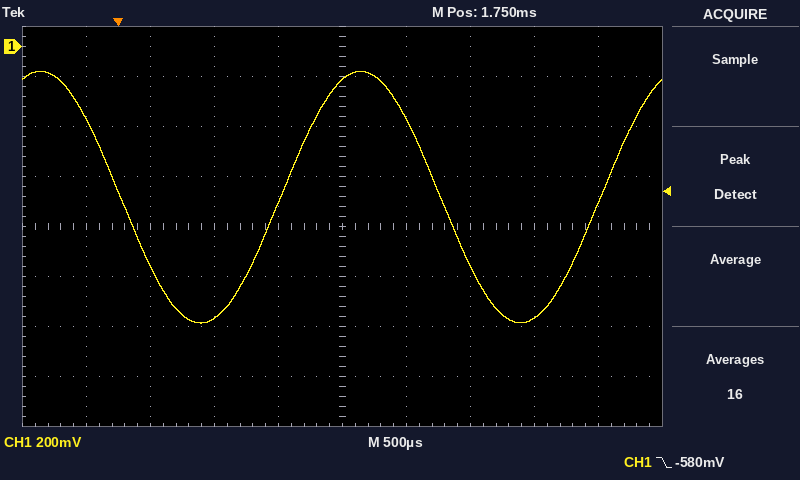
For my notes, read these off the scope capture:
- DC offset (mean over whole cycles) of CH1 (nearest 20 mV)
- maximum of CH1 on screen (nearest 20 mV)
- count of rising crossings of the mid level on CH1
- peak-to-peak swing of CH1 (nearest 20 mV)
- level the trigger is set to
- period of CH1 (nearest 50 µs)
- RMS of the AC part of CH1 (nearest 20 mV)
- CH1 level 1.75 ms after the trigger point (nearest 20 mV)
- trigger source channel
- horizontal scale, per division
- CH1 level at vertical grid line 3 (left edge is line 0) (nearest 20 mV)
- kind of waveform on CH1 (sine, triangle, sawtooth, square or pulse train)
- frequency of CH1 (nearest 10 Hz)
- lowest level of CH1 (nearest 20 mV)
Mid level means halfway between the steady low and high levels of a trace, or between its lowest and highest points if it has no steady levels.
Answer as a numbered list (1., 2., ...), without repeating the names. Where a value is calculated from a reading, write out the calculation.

1. (-100 mV + (-1.10 V)) / 2 ≈ -600 mV
2. -100 mV
3. 2
4. -100 mV − (-1.10 V) = 1.00 V
5. -580 mV
6. 2.50 ms
7. 1.00 V / (2√2) ≈ 354 mV, so 360 mV to the nearest 20 mV
8. -140 mV
9. CH1
10. 500 µs
11. -1.08 V
12. sine
13. 1 / 2.50 ms ≈ 400 Hz
14. -1.10 V
